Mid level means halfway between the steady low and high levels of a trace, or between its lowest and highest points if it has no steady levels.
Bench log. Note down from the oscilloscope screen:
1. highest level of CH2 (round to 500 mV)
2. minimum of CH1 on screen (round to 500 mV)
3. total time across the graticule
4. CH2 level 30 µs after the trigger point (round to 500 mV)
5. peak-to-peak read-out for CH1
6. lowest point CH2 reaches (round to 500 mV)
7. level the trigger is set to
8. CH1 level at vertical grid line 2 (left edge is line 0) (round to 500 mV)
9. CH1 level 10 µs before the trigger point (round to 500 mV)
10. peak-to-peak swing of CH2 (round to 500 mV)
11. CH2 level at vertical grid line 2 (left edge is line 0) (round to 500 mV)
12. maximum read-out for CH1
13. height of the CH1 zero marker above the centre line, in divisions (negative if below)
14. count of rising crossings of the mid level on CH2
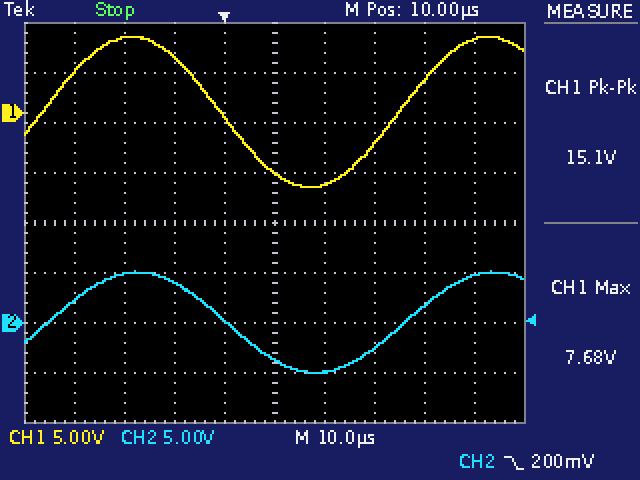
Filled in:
5.0 V
-7.5 V
100 µs
-2.5 V
15.1 V
-5.0 V
200 mV
7.5 V
5.5 V
10.0 V
5.0 V
7.68 V
+2.2 div
2
